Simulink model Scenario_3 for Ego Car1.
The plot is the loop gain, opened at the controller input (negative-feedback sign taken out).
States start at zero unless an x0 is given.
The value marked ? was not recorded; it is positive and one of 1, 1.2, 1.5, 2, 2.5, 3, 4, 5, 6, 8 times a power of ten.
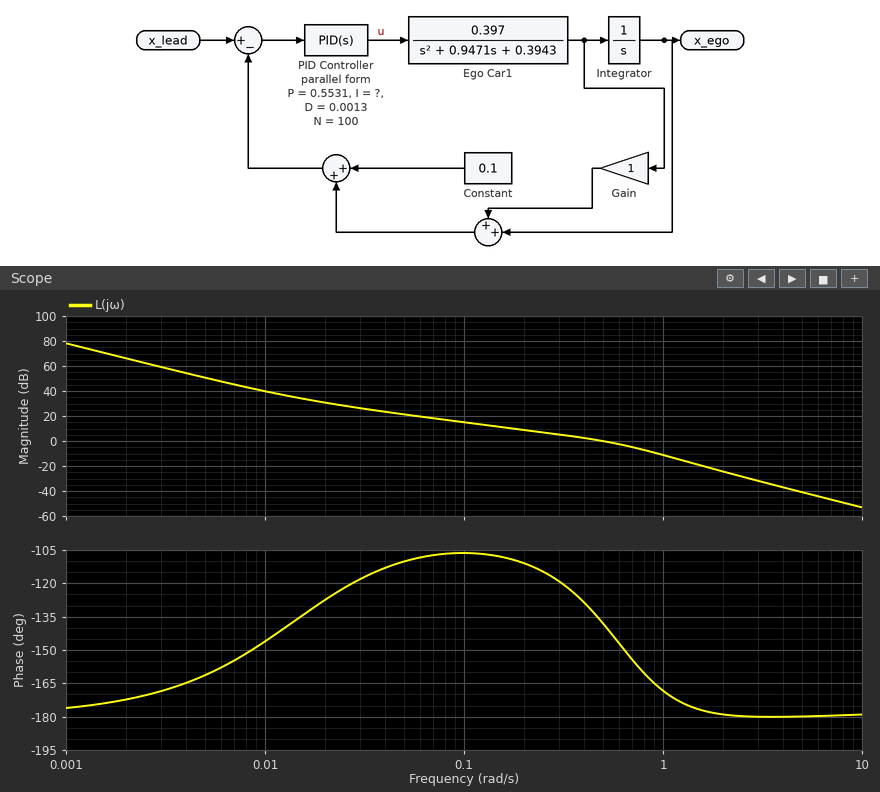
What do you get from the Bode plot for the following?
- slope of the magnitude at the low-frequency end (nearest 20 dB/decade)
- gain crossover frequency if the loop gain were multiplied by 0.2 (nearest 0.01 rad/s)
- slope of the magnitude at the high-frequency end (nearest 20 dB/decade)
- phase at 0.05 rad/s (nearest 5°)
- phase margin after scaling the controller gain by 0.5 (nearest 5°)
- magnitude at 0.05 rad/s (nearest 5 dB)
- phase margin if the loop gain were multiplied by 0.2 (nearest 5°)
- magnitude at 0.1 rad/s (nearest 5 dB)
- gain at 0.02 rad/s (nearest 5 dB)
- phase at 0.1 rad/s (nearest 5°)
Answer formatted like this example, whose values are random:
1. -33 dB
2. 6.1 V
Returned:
1. -40 dB/decade
2. 0.11 rad/s
3. -40 dB/decade
4. -110°
5. 65°
6. 20 dB
7. 75°
8. 15 dB
9. 30 dB
10. -105°
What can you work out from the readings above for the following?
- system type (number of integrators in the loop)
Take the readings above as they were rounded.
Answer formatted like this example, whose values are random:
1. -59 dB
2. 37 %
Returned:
1. 2
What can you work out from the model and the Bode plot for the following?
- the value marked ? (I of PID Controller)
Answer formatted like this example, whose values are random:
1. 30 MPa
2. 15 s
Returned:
1. 0.008
